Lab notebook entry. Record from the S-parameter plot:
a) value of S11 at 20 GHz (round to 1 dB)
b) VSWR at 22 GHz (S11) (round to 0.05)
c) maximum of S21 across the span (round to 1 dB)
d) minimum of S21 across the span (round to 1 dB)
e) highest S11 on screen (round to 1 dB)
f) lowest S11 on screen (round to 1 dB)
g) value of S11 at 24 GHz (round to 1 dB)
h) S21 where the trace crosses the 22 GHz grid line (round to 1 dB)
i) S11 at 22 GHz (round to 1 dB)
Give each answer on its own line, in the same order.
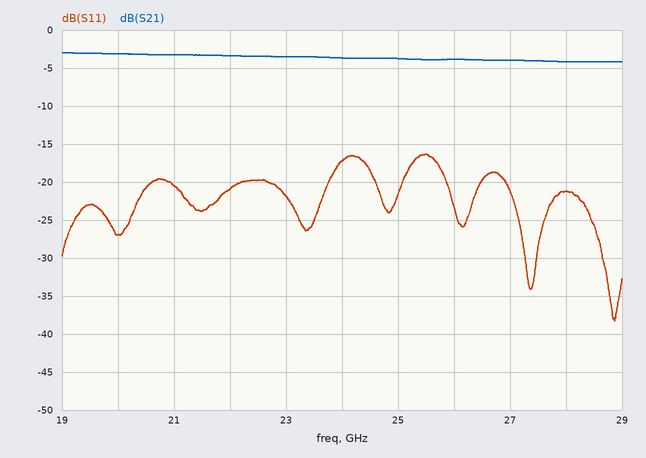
-27 dB
1.20
-3 dB
-4 dB
-16 dB
-38 dB
-17 dB
-3 dB
-21 dB
